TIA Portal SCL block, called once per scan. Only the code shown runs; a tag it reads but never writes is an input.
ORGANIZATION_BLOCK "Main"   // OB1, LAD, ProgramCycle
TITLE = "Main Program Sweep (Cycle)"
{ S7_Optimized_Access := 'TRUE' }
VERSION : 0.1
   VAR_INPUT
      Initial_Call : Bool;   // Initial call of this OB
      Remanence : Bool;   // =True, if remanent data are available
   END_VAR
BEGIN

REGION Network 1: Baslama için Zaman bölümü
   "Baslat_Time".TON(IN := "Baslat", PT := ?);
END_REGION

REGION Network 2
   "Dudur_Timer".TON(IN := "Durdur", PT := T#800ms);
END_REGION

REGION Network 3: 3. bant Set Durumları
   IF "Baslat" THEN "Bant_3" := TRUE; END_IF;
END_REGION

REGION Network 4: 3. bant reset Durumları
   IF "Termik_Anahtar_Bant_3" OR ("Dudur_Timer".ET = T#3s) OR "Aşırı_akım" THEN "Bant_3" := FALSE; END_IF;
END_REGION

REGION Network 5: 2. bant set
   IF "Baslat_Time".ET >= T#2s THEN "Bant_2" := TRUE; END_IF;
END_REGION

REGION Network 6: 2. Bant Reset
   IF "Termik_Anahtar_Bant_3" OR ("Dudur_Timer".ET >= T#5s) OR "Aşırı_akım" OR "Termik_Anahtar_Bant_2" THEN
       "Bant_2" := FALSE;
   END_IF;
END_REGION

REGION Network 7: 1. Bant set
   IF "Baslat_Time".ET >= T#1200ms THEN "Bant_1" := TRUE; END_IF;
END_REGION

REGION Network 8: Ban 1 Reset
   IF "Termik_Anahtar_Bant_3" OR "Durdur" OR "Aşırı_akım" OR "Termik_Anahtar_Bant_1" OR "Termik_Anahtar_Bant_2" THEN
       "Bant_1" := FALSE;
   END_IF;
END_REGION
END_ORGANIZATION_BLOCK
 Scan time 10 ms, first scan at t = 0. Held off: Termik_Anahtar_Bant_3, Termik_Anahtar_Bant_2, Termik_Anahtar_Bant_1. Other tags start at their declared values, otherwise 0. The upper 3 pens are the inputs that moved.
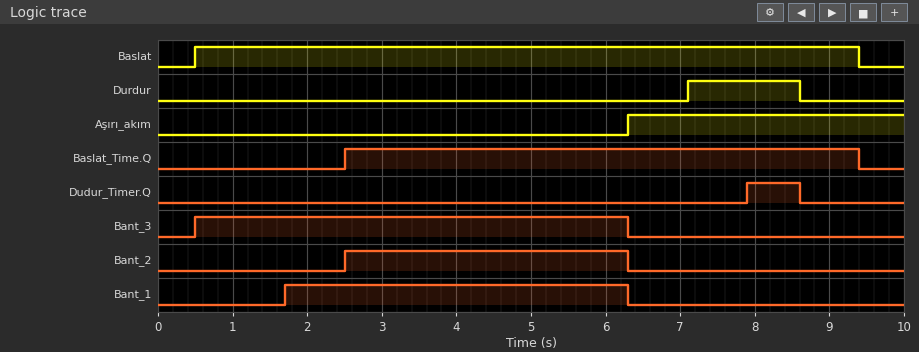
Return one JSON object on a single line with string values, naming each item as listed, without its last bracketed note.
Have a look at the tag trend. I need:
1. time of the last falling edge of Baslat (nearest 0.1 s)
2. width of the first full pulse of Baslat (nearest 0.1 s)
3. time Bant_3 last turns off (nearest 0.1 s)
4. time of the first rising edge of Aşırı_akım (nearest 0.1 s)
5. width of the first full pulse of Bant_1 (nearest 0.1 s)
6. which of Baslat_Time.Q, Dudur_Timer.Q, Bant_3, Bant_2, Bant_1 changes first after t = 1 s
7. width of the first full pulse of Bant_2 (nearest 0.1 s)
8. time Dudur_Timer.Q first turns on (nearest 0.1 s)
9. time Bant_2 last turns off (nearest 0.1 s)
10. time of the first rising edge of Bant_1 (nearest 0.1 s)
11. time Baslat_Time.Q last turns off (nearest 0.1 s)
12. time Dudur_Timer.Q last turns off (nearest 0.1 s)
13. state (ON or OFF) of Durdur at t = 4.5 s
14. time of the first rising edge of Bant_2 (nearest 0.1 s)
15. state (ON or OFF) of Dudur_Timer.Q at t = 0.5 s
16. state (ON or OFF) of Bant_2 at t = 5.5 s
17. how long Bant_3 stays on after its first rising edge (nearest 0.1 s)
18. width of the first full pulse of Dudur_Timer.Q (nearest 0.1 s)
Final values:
{"time of the last falling edge of Baslat": "9.4 s", "width of the first full pulse of Baslat": "8.9 s", "time Bant_3 last turns off": "6.3 s", "time of the first rising edge of Aşırı_akım": "6.3 s", "width of the first full pulse of Bant_1": "4.6 s", "which of Baslat_Time.Q, Dudur_Timer.Q, Bant_3, Bant_2, Bant_1 changes first after t = 1 s": "Bant_1", "width of the first full pulse of Bant_2": "3.8 s", "time Dudur_Timer.Q first turns on": "7.9 s", "time Bant_2 last turns off": "6.3 s", "time of the first rising edge of Bant_1": "1.7 s", "time Baslat_Time.Q last turns off": "9.4 s", "time Dudur_Timer.Q last turns off": "8.6 s", "state (ON or OFF) of Durdur at t = 4.5 s": "OFF", "time of the first rising edge of Bant_2": "2.5 s", "state (ON or OFF) of Dudur_Timer.Q at t = 0.5 s": "OFF", "state (ON or OFF) of Bant_2 at t = 5.5 s": "ON", "how long Bant_3 stays on after its first rising edge": "5.8 s", "width of the first full pulse of Dudur_Timer.Q": "0.7 s"}
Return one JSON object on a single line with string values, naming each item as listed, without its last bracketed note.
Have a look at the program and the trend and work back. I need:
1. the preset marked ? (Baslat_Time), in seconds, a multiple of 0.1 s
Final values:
{"the preset marked ? (Baslat_Time), in seconds, a multiple of 0.1 s": "2.0 s"}
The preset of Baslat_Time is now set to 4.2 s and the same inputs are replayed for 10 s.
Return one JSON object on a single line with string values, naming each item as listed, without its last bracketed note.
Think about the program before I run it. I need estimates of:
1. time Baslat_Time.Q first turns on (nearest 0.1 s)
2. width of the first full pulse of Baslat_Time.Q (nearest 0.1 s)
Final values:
{"time Baslat_Time.Q first turns on": "4.7 s", "width of the first full pulse of Baslat_Time.Q": "4.7 s"}
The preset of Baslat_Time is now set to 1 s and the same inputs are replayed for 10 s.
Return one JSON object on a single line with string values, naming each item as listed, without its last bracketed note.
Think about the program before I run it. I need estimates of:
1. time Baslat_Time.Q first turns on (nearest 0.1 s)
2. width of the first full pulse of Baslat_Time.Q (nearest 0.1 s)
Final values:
{"time Baslat_Time.Q first turns on": "1.5 s", "width of the first full pulse of Baslat_Time.Q": "7.9 s"}
